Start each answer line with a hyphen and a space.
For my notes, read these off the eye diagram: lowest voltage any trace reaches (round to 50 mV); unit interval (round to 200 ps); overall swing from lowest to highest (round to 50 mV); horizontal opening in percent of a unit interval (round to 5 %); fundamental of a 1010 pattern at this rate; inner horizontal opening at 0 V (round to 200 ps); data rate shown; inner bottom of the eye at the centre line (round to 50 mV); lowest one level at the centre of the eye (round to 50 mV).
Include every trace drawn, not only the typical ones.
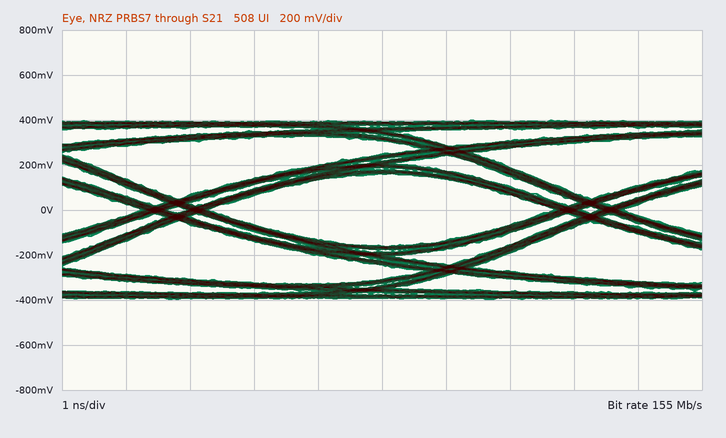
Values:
- -400 mV
- 6.4 ns
- 800 mV
- 85 %
- 77.5 MHz
- 5.4 ns
- 155 Mb/s
- -150 mV
- 150 mV
